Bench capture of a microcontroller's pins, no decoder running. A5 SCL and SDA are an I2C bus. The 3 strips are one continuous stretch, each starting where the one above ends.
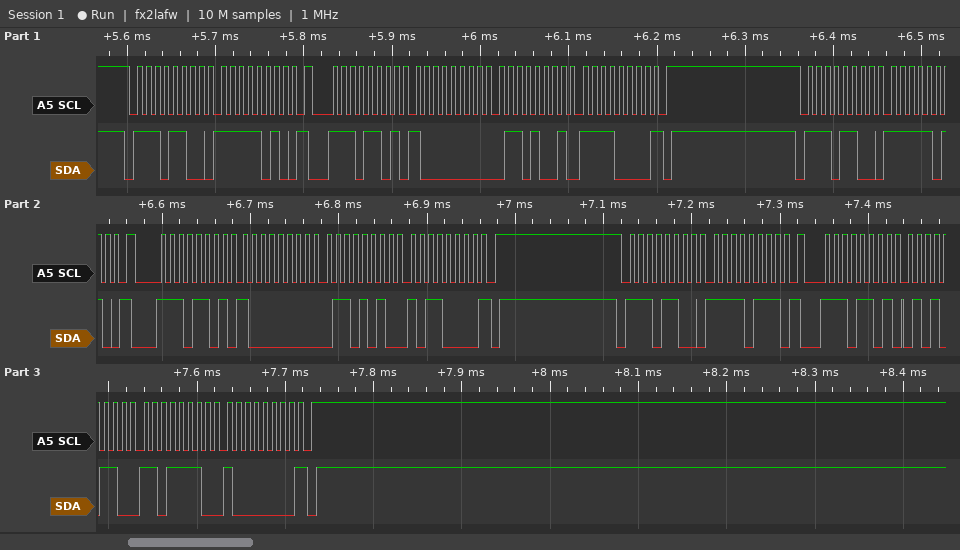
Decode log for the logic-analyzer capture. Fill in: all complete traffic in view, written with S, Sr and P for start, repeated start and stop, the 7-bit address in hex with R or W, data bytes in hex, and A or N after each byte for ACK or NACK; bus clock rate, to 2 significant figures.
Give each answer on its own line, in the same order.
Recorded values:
S 76W A FA A Sr 76R A 80 A 69 A F0 N P S 76W A FA A Sr 76R A 80 A 6A A B0 N P S 76W A F7 A Sr 76R A 56 A DE A 80 N P
100 kHz
